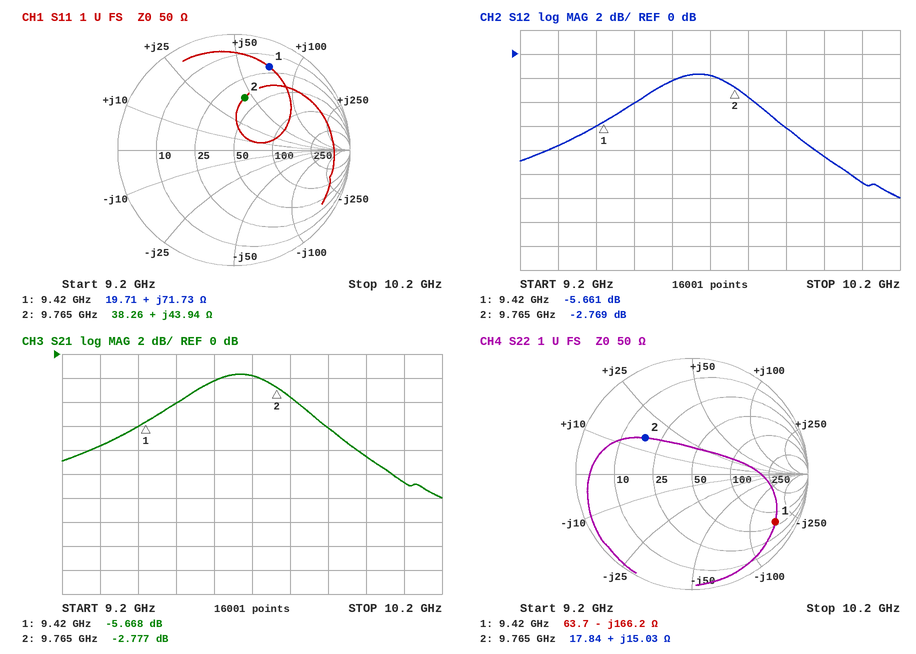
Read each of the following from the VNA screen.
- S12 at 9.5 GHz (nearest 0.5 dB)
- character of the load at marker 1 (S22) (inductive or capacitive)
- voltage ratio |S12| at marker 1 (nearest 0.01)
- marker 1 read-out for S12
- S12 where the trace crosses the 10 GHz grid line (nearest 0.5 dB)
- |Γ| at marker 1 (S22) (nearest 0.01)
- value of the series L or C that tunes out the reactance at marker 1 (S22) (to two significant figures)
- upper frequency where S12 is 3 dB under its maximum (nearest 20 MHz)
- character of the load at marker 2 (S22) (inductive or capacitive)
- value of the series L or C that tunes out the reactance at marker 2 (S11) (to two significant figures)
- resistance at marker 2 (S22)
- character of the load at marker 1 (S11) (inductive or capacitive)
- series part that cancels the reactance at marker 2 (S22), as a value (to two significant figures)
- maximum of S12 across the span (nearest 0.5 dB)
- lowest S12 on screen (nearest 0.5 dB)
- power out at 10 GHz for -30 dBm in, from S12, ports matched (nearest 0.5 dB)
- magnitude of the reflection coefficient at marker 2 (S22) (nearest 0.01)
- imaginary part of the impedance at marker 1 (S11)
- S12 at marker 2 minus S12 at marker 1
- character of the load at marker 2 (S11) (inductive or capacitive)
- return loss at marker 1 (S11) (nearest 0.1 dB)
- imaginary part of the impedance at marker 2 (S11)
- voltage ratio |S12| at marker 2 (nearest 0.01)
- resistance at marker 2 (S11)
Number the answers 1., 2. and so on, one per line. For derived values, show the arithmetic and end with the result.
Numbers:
1. -4.0 dB
2. capacitive
3. 10^(-5.661/20) ≈ 0.52
4. -5.661 dB
5. -8.5 dB
6. 0.83
7. L = 166.2 Ω/(2π × 9.42 GHz) ≈ 2.8 nH
8. 9.84 GHz
9. inductive
10. C = 1/(2π × 9.765 GHz × 43.94 Ω) ≈ 371 fF, so 370 fF to two significant figures
11. 17.84 Ω
12. inductive
13. C = 1/(2π × 9.765 GHz × 15.03 Ω) ≈ 1.1 pF
14. -1.5 dB
15. -12.0 dB
16. -30 dBm + (-8.5 dB) = -38.5 dBm
17. 0.51
18. +71.73 Ω
19. -2.769 − (-5.661) = 2.892 dB
20. inductive
21. 2.2 dB
22. +43.94 Ω
23. 10^(-2.769/20) ≈ 0.73
24. 38.26 Ω
